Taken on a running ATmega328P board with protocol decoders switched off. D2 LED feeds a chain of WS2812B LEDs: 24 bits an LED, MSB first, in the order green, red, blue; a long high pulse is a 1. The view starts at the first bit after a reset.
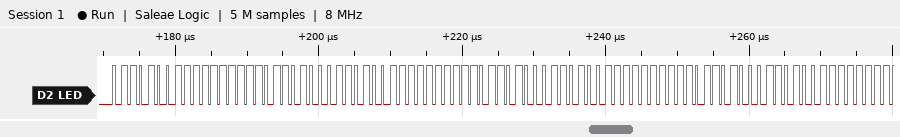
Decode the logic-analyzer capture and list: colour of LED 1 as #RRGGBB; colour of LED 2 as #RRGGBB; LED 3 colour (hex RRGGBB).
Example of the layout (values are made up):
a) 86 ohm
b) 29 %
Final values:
a) #FF69B4
b) #FF69B4
c) #FF69B4
